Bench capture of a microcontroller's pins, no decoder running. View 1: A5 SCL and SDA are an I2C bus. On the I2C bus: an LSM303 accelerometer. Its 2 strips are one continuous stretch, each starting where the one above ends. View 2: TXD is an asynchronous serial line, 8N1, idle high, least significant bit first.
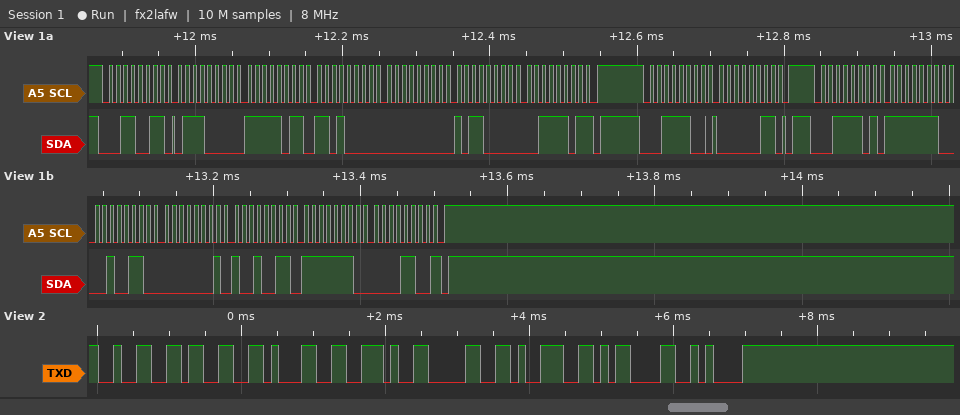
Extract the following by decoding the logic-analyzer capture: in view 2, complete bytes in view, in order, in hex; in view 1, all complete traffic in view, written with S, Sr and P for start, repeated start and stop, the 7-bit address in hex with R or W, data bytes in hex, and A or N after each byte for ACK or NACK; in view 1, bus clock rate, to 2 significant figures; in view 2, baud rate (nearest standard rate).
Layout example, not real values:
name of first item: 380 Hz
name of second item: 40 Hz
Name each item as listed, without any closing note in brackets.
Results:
in view 2, complete bytes in view, in order, in hex: 32 33 31 2E 30 39 0D 0A
in view 1, all complete traffic in view, written with S, Sr and P for start, repeated start and stop, the 7-bit address in hex with R or W, data bytes in hex, and A or N after each byte for ACK or NACK: S 19R A 70 A FB A D0 A 00 A B0 A 3D N P S 1EW A 03 A P S 1ER A FE A 26 A 01 A 93 A FE A 0C N P
in view 1, bus clock rate, to 2 significant figures: 100 kHz
in view 2, baud rate: 9600 baud
